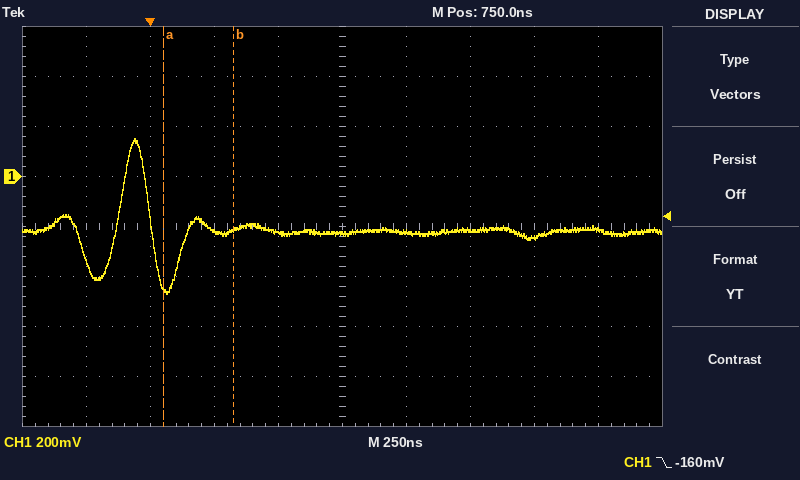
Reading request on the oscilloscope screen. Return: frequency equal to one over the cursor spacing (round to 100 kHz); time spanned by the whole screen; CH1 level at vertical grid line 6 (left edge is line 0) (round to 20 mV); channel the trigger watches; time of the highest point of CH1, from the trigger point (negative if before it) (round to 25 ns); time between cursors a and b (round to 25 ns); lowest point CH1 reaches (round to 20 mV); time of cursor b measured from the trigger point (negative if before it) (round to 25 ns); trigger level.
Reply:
3.6 MHz
2.5 µs
-220 mV
CH1
-50 ns
275 ns
-460 mV
+325 ns
-160 mV
